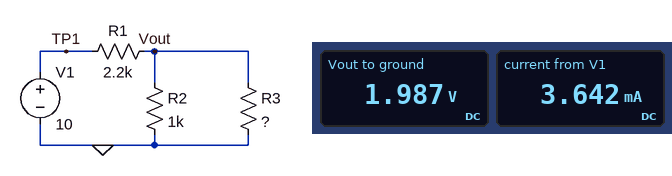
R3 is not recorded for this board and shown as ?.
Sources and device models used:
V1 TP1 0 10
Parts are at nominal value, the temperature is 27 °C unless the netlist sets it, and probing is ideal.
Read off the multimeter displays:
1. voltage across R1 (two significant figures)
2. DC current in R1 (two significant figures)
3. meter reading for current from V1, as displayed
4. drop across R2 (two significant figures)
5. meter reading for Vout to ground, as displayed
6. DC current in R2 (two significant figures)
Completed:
8.0 V
3.6 mA
3.642 mA
2.0 V
1.987 V
2.0 mA
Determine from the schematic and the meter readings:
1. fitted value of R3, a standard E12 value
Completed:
1.2 kΩ
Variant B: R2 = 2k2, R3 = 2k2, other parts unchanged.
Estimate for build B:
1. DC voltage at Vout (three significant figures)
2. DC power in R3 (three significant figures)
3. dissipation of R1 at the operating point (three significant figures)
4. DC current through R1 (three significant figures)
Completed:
3.33 V
5.05 mW
20.2 mW
3.03 mA
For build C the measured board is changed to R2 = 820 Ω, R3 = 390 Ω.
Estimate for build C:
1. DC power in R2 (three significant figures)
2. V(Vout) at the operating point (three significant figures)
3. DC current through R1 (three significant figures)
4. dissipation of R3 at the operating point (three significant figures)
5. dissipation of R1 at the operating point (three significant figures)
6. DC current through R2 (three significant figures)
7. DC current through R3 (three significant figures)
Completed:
1.40 mW
1.07 V
4.06 mA
2.95 mW
36.2 mW
1.31 mA
2.75 mA
